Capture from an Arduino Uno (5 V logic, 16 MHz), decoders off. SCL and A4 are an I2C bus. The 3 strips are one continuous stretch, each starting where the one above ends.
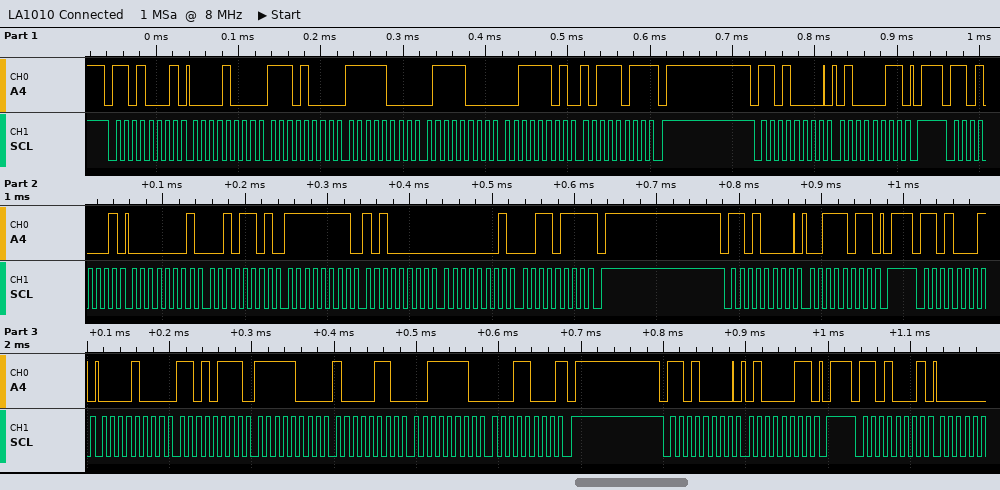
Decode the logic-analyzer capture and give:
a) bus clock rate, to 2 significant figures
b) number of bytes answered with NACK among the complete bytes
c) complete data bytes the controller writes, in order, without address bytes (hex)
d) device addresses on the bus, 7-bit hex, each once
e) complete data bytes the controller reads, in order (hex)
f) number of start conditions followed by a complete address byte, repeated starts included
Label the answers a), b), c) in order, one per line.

a) 100 kHz
b) 3
c) 43 3B 43
d) 0x68
e) 08 E8 F8 78 3D BB 01 2D FF A0 01 37 08 D7 F8 86 3E 18
f) 7
